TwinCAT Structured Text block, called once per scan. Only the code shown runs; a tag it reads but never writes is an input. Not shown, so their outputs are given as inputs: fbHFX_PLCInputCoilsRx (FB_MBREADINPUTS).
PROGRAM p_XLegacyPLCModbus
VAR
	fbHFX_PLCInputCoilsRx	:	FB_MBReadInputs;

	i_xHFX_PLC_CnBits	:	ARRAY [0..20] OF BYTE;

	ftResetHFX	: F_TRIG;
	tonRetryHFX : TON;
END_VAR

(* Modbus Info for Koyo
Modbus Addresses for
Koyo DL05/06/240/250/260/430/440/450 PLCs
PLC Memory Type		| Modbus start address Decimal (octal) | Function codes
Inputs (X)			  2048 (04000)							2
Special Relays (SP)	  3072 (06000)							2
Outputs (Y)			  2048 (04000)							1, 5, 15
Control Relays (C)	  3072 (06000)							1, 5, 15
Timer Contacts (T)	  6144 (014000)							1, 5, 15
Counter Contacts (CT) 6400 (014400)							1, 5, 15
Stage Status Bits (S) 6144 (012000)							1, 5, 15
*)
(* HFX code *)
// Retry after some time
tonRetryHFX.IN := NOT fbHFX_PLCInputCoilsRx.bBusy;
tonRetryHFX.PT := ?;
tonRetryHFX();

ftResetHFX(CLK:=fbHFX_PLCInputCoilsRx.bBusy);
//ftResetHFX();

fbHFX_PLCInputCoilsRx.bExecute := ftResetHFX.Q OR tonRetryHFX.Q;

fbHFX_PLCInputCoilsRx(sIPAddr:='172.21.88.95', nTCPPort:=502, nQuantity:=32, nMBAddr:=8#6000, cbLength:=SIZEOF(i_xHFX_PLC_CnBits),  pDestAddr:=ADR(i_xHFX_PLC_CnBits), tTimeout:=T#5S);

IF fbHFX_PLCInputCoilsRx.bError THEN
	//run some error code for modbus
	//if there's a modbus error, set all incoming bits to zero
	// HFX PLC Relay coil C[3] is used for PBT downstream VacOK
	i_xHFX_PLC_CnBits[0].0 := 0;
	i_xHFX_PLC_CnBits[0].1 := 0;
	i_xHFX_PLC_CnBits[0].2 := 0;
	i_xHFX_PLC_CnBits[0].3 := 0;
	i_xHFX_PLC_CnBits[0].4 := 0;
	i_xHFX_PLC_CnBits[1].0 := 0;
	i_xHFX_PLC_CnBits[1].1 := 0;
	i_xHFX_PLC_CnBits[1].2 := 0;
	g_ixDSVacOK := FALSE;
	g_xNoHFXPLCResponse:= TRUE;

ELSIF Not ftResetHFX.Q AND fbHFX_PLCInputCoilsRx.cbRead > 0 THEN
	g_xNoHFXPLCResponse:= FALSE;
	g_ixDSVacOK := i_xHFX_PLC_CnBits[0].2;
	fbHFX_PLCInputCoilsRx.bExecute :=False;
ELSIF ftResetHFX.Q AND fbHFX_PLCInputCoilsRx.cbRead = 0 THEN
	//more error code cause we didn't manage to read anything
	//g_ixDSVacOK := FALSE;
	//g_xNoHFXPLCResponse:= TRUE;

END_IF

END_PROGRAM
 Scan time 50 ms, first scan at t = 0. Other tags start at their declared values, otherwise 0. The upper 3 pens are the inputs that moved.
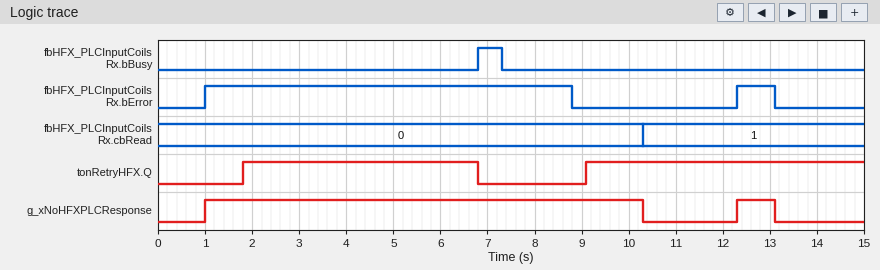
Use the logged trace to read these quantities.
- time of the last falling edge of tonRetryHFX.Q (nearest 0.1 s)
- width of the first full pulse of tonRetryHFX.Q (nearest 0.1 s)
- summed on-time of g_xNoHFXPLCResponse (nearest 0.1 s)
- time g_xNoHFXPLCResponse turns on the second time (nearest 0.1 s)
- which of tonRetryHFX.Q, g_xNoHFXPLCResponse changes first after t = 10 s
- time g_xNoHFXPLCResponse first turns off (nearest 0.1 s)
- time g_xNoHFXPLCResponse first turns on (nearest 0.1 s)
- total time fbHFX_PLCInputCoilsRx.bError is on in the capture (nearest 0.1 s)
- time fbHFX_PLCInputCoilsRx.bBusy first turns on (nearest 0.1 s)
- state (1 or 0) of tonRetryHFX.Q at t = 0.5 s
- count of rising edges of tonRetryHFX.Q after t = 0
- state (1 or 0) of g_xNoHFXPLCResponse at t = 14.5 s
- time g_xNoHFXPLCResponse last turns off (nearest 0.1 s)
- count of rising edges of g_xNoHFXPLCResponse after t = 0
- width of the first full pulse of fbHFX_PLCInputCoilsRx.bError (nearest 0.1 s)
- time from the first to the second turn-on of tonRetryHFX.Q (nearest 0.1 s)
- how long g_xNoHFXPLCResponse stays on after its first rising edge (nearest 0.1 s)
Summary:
6.8 s
5.0 s
10.1 s
12.3 s
g_xNoHFXPLCResponse
10.3 s
1.0 s
8.6 s
6.8 s
0
2
0
13.1 s
2
7.8 s
7.3 s
9.3 s
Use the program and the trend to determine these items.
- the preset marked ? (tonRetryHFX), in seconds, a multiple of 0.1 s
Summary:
1.8 s
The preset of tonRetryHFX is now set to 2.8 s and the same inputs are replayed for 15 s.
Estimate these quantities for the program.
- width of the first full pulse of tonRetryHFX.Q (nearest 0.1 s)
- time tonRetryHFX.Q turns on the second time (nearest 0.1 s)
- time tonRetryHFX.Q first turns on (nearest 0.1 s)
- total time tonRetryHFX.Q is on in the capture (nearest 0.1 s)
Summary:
4.0 s
10.1 s
2.8 s
8.9 s
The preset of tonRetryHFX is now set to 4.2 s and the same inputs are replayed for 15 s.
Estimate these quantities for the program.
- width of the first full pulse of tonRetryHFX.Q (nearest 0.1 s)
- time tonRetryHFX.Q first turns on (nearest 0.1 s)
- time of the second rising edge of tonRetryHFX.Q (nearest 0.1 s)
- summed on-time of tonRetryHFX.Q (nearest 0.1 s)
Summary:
2.6 s
4.2 s
11.5 s
6.1 s
